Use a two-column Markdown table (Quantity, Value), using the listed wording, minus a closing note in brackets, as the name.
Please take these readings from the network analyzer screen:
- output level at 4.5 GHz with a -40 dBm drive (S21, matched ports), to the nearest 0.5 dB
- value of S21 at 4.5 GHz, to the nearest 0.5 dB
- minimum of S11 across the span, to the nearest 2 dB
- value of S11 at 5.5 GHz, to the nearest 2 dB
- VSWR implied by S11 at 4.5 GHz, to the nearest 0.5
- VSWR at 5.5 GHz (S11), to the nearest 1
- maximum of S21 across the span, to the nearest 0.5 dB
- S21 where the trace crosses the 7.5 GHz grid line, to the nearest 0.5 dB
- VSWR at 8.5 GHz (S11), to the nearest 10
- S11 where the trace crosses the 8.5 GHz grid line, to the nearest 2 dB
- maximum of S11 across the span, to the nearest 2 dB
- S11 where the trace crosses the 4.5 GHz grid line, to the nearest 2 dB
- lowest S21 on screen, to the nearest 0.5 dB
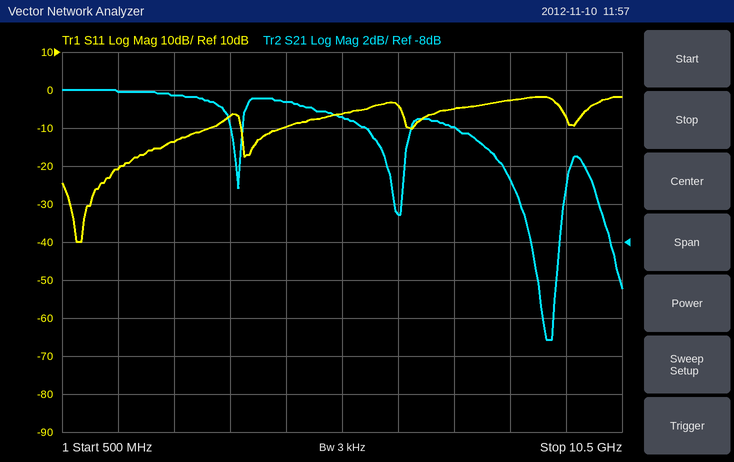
| Quantity | Value |
|---|---|
| output level at 4.5 GHz with a -40 dBm drive (S21, matched ports), to the nearest 0.5 dB | -40.5 dBm |
| value of S21 at 4.5 GHz, to the nearest 0.5 dB | -0.5 dB |
| minimum of S11 across the span, to the nearest 2 dB | -40 dB |
| value of S11 at 5.5 GHz, to the nearest 2 dB | -6 dB |
| VSWR implied by S11 at 4.5 GHz, to the nearest 0.5 | 2.0 |
| VSWR at 5.5 GHz (S11), to the nearest 1 | 3 |
| maximum of S21 across the span, to the nearest 0.5 dB | 0.0 dB |
| S21 where the trace crosses the 7.5 GHz grid line, to the nearest 0.5 dB | -2.0 dB |
| VSWR at 8.5 GHz (S11), to the nearest 10 | 10 |
| S11 where the trace crosses the 8.5 GHz grid line, to the nearest 2 dB | -2 dB |
| maximum of S11 across the span, to the nearest 2 dB | -2 dB |
| S11 where the trace crosses the 4.5 GHz grid line, to the nearest 2 dB | -10 dB |
| lowest S21 on screen, to the nearest 0.5 dB | -13.0 dB |
